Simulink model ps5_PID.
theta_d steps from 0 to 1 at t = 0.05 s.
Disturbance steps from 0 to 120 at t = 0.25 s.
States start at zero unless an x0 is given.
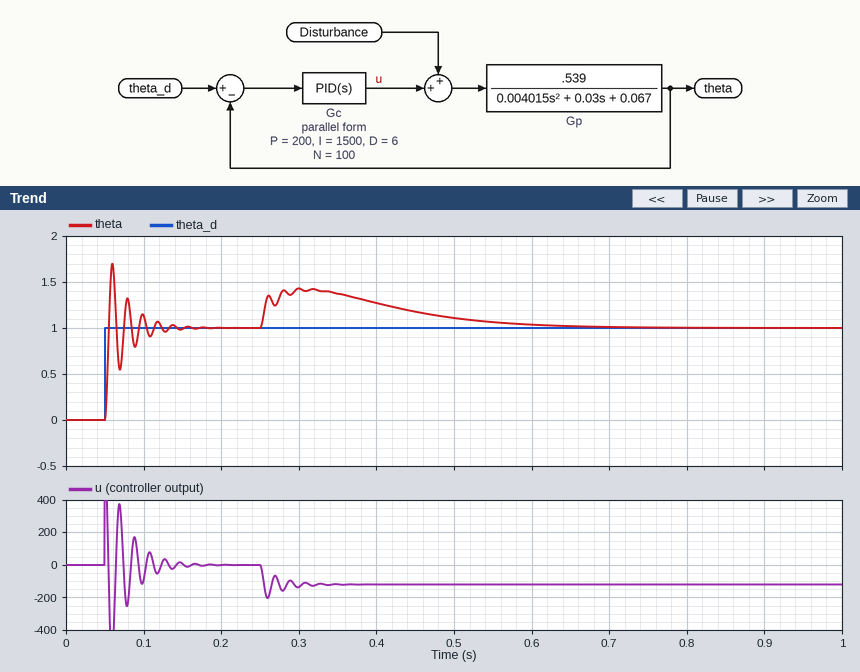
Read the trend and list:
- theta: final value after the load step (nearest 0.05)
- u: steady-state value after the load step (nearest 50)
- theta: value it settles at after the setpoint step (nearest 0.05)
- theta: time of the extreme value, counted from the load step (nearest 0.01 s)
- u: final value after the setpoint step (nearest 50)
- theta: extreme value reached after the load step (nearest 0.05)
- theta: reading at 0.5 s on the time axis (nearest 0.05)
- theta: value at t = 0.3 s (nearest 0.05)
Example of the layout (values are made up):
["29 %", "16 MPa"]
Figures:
["1.00", "-100", "1.00", "0.05 s", "0", "1.45", "1.10", "1.45"]
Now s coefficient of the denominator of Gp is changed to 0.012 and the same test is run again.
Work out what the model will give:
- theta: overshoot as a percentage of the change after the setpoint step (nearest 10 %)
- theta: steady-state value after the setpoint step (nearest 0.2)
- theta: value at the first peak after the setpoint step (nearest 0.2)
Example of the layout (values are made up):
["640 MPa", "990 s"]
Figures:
["70 %", "1.0", "1.8"]
